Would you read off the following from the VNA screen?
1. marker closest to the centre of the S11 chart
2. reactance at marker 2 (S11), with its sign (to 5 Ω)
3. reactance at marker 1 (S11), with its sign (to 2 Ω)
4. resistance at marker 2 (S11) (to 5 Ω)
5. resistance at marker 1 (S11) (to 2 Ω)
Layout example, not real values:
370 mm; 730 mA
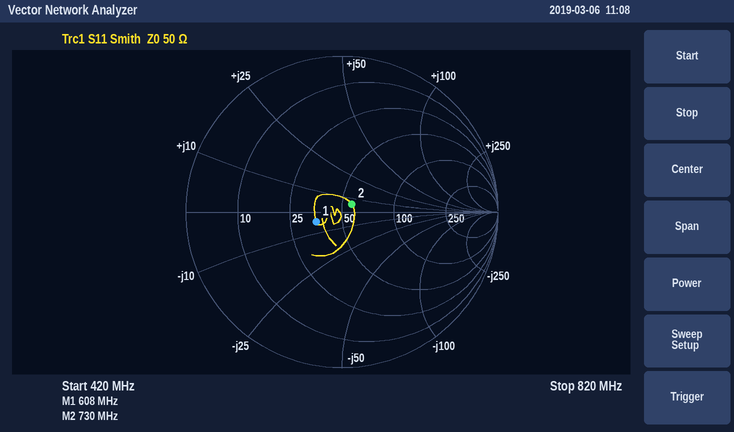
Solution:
marker 2; +5 Ω; -4 Ω; 55 Ω; 36 Ω
